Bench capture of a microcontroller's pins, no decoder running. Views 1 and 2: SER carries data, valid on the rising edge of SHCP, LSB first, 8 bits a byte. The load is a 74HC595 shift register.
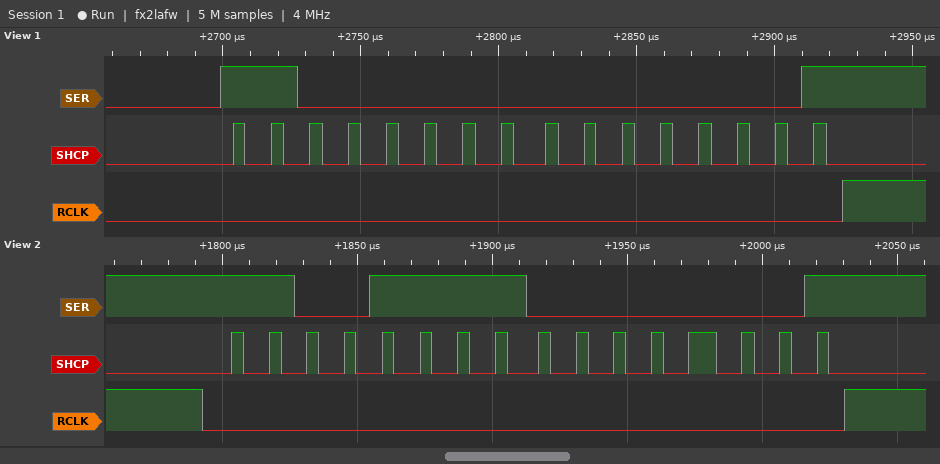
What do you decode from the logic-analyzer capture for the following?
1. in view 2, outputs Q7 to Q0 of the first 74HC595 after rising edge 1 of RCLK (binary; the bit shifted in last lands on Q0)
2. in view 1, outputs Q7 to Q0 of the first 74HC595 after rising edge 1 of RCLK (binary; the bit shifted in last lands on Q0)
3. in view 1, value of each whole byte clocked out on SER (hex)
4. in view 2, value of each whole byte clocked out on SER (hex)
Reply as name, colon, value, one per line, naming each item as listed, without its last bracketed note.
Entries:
in view 2, outputs Q7 to Q0 of the first 74HC595 after rising edge 1 of RCLK: 00000001
in view 1, outputs Q7 to Q0 of the first 74HC595 after rising edge 1 of RCLK: 00000001
in view 1, value of each whole byte clocked out on SER: 03 80
in view 2, value of each whole byte clocked out on SER: F3 80
